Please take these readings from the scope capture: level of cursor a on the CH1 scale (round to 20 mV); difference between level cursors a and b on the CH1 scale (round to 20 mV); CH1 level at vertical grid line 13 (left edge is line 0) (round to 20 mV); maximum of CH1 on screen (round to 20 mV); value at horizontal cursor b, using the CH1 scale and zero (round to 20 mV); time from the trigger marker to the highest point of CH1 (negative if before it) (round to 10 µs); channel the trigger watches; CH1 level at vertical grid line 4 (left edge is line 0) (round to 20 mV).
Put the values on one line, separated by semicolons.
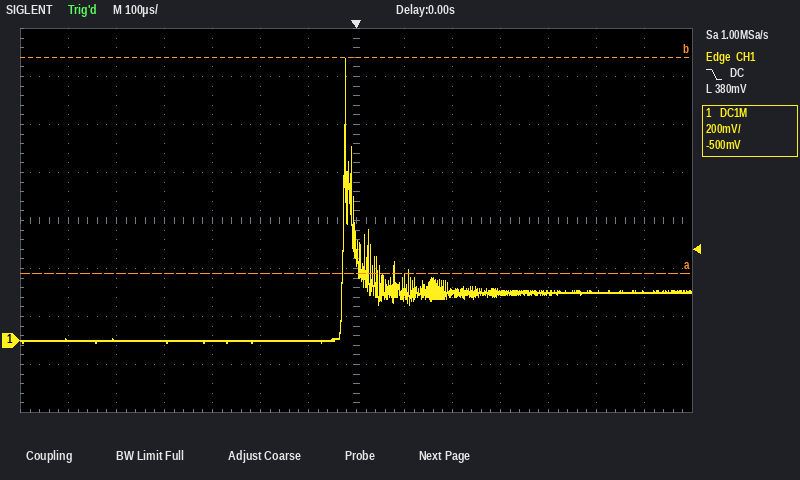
280 mV; 900 mV; 200 mV; 1.18 V; 1.18 V; -20 µs; CH1; 0 mV
